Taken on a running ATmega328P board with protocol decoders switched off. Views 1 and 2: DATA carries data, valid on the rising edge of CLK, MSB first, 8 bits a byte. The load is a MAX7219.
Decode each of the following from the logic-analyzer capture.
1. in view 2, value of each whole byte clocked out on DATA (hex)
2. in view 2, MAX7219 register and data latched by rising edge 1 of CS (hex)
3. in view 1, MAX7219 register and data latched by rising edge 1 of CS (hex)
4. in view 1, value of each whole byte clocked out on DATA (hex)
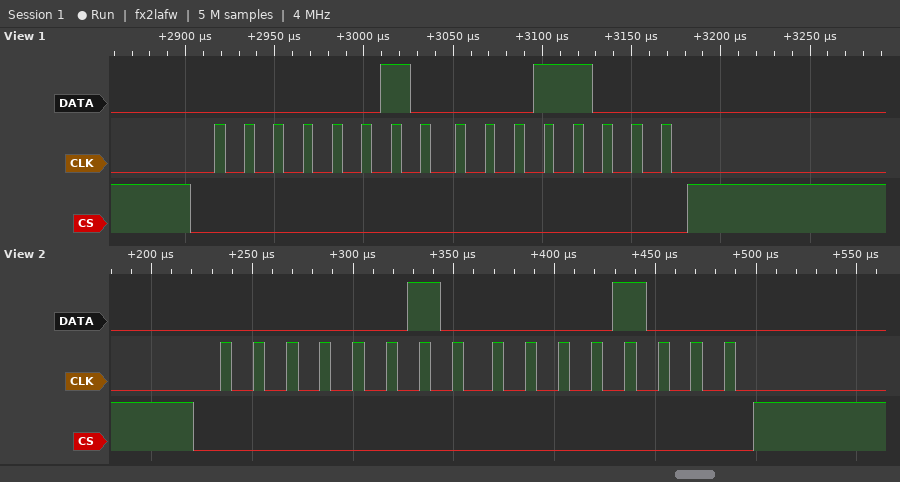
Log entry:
02 08
register 0x2, data 0x08
register 0x2, data 0x18
0x02 0x18
